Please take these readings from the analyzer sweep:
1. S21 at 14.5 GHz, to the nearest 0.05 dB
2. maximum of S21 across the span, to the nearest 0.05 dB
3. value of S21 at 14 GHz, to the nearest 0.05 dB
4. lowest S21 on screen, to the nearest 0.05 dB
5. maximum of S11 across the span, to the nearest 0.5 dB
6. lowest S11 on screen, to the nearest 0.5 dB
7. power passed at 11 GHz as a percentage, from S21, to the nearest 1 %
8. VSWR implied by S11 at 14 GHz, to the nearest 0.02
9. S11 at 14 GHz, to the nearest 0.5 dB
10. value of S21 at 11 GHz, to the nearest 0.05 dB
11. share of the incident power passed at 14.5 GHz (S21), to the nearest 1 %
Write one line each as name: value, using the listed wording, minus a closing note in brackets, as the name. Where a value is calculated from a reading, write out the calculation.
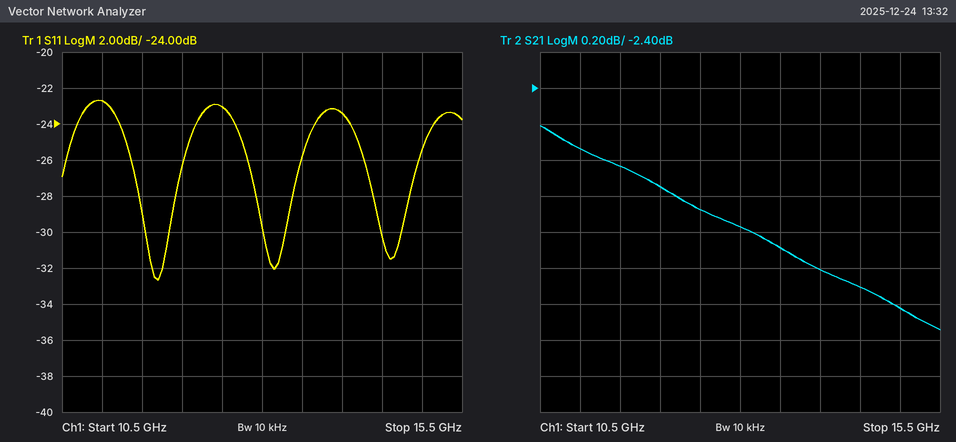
S21 at 14.5 GHz, to the nearest 0.05 dB: -3.50 dB
maximum of S21 across the span, to the nearest 0.05 dB: -2.60 dB
value of S21 at 14 GHz, to the nearest 0.05 dB: -3.40 dB
lowest S21 on screen, to the nearest 0.05 dB: -3.75 dB
maximum of S11 across the span, to the nearest 0.5 dB: -22.5 dB
lowest S11 on screen, to the nearest 0.5 dB: -32.5 dB
power passed at 11 GHz as a percentage, from S21, to the nearest 1 %: 10^(-2.75/10) ≈ 53 %
VSWR implied by S11 at 14 GHz, to the nearest 0.02: |Γ| = 10^(-23.5/20) = 0.0668; VSWR = (1 + 0.0668)/(1 − 0.0668) ≈ 1.14
S11 at 14 GHz, to the nearest 0.5 dB: -23.5 dB
value of S21 at 11 GHz, to the nearest 0.05 dB: -2.75 dB
share of the incident power passed at 14.5 GHz (S21), to the nearest 1 %: 10^(-3.5/10) ≈ 45 %
